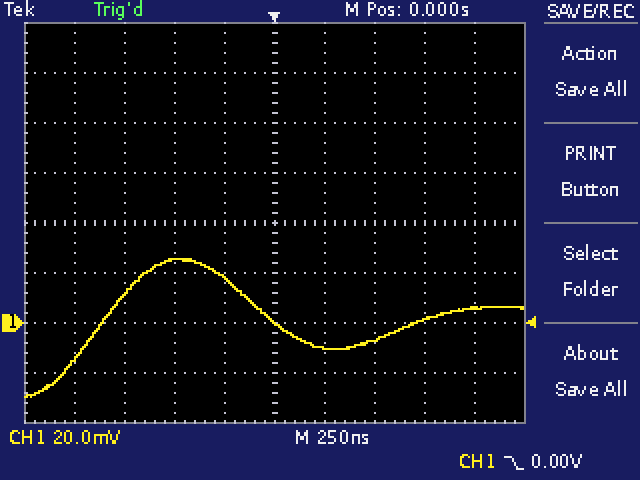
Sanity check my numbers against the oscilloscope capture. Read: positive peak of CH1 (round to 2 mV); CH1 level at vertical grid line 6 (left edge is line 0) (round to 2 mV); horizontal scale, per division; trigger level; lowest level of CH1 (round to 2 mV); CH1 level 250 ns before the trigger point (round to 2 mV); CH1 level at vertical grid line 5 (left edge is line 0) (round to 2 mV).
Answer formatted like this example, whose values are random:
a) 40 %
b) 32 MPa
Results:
a) 26 mV
b) -10 mV
c) 250 ns
d) 0.00 V
e) -30 mV
f) 18 mV
g) 0 mV
